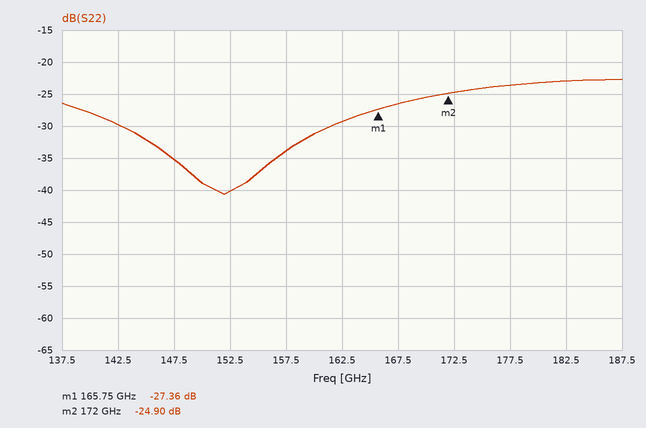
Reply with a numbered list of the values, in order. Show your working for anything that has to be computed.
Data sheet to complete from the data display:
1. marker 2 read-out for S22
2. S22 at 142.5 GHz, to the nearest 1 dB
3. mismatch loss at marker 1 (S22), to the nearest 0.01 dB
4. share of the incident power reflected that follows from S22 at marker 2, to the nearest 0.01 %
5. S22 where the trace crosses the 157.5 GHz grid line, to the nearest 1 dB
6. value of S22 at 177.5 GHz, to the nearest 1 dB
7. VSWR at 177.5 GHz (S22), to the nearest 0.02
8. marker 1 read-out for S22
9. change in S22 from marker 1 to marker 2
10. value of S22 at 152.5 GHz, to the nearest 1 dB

1. -24.90 dB
2. -30 dB
3. −10 log10(1 − 10^(-27.36/10)) ≈ 0.01 dB
4. 10^(-24.9/10) ≈ 0.32 %
5. -34 dB
6. -24 dB
7. |Γ| = 10^(-24/20) = 0.0631; VSWR = (1 + 0.0631)/(1 − 0.0631) ≈ 1.13, so 1.14 to the nearest 0.02
8. -27.36 dB
9. -24.9 − (-27.36) = 2.46 dB
10. -40 dB
